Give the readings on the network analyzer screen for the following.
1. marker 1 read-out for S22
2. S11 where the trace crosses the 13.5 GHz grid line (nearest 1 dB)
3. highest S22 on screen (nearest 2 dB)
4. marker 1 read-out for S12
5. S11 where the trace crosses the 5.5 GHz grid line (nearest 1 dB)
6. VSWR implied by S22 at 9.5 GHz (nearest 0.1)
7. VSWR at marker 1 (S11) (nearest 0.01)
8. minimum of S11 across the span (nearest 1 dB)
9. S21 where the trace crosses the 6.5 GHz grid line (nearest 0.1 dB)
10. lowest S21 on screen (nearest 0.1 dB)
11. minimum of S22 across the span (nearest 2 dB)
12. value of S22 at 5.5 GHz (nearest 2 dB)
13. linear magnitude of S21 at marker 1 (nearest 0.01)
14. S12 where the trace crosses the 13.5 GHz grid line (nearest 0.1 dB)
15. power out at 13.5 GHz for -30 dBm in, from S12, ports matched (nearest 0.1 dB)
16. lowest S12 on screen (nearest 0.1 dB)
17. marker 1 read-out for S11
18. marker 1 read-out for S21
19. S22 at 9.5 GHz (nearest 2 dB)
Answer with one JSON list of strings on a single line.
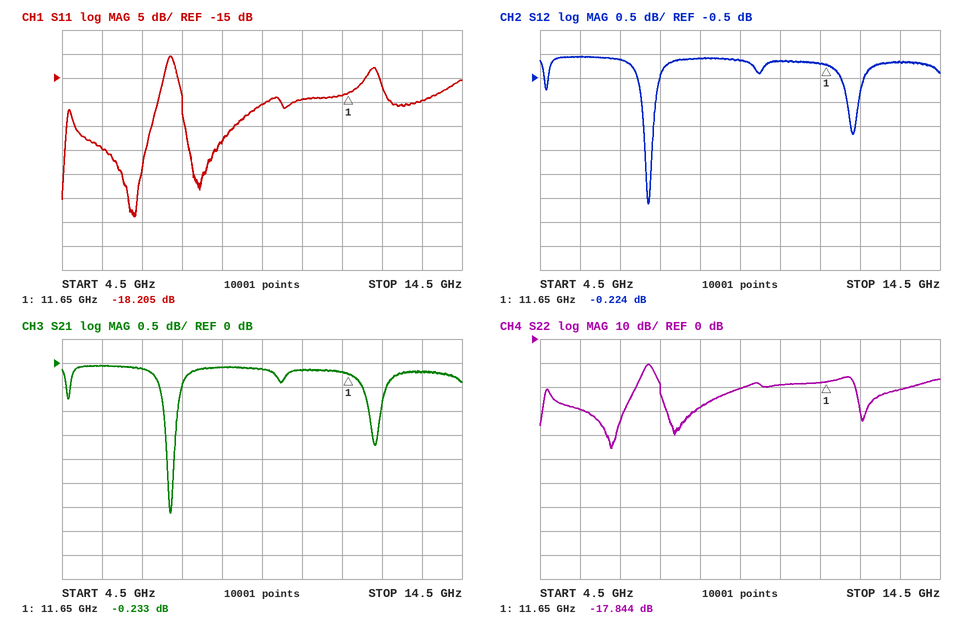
["-17.844 dB", "-20 dB", "-10 dB", "-0.224 dB", "-30 dB", "1.2", "1.28", "-44 dB", "-0.1 dB", "-3.1 dB", "-46 dB", "-30 dB", "0.97", "-0.2 dB", "-30.2 dBm", "-3.1 dB", "-18.205 dB", "-0.233 dB", "-20 dB"]
